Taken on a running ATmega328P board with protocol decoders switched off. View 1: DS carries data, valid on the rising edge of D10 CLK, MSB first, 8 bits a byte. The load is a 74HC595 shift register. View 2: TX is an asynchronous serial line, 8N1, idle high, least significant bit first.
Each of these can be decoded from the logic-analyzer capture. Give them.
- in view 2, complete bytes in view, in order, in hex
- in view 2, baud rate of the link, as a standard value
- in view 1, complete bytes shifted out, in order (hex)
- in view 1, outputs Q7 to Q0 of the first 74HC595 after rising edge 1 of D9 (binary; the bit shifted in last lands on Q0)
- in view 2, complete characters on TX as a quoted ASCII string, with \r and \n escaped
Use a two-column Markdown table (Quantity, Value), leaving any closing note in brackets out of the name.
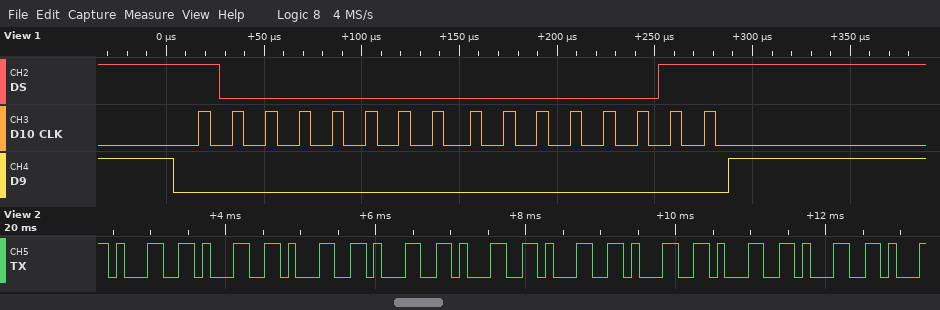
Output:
| Quantity | Value |
|---|---|
| in view 2, complete bytes in view, in order, in hex | 31 31 31 31 31 31 31 31 31 |
| in view 2, baud rate of the link, as a standard value | 9600 baud |
| in view 1, complete bytes shifted out, in order | 0x80 0x03 |
| in view 1, outputs Q7 to Q0 of the first 74HC595 after rising edge 1 of D9 | 00000011 |
| in view 2, complete characters on TX as a quoted ASCII string, with \r and \n escaped | "111111111" |
